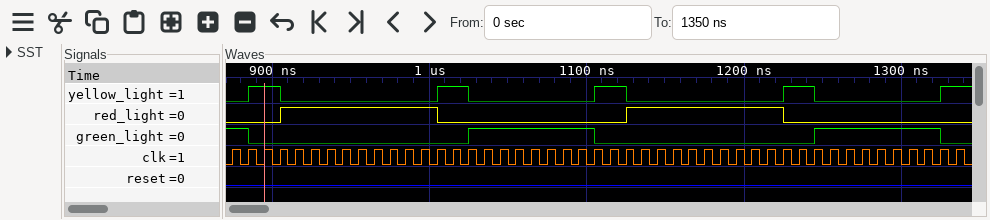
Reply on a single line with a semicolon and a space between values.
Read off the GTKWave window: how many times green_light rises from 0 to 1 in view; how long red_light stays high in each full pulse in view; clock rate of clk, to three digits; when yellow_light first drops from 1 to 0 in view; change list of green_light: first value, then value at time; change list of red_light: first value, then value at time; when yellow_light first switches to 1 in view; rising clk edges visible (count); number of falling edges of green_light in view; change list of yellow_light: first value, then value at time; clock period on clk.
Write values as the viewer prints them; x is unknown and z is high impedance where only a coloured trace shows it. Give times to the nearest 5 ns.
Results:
2; 100 ns, 100 ns; 100 MHz; 905 ns; 1, 0 at 885 ns, 1 at 1025 ns, 0 at 1105 ns, 1 at 1245 ns, 0 at 1325 ns; 0, 1 at 905 ns, 0 at 1005 ns, 1 at 1125 ns, 0 at 1225 ns; 885 ns; 47; 3; 0, 1 at 885 ns, 0 at 905 ns, 1 at 1005 ns, 0 at 1025 ns, 1 at 1105 ns, 0 at 1125 ns, 1 at 1225 ns, 0 at 1245 ns, 1 at 1325 ns; 10 ns
